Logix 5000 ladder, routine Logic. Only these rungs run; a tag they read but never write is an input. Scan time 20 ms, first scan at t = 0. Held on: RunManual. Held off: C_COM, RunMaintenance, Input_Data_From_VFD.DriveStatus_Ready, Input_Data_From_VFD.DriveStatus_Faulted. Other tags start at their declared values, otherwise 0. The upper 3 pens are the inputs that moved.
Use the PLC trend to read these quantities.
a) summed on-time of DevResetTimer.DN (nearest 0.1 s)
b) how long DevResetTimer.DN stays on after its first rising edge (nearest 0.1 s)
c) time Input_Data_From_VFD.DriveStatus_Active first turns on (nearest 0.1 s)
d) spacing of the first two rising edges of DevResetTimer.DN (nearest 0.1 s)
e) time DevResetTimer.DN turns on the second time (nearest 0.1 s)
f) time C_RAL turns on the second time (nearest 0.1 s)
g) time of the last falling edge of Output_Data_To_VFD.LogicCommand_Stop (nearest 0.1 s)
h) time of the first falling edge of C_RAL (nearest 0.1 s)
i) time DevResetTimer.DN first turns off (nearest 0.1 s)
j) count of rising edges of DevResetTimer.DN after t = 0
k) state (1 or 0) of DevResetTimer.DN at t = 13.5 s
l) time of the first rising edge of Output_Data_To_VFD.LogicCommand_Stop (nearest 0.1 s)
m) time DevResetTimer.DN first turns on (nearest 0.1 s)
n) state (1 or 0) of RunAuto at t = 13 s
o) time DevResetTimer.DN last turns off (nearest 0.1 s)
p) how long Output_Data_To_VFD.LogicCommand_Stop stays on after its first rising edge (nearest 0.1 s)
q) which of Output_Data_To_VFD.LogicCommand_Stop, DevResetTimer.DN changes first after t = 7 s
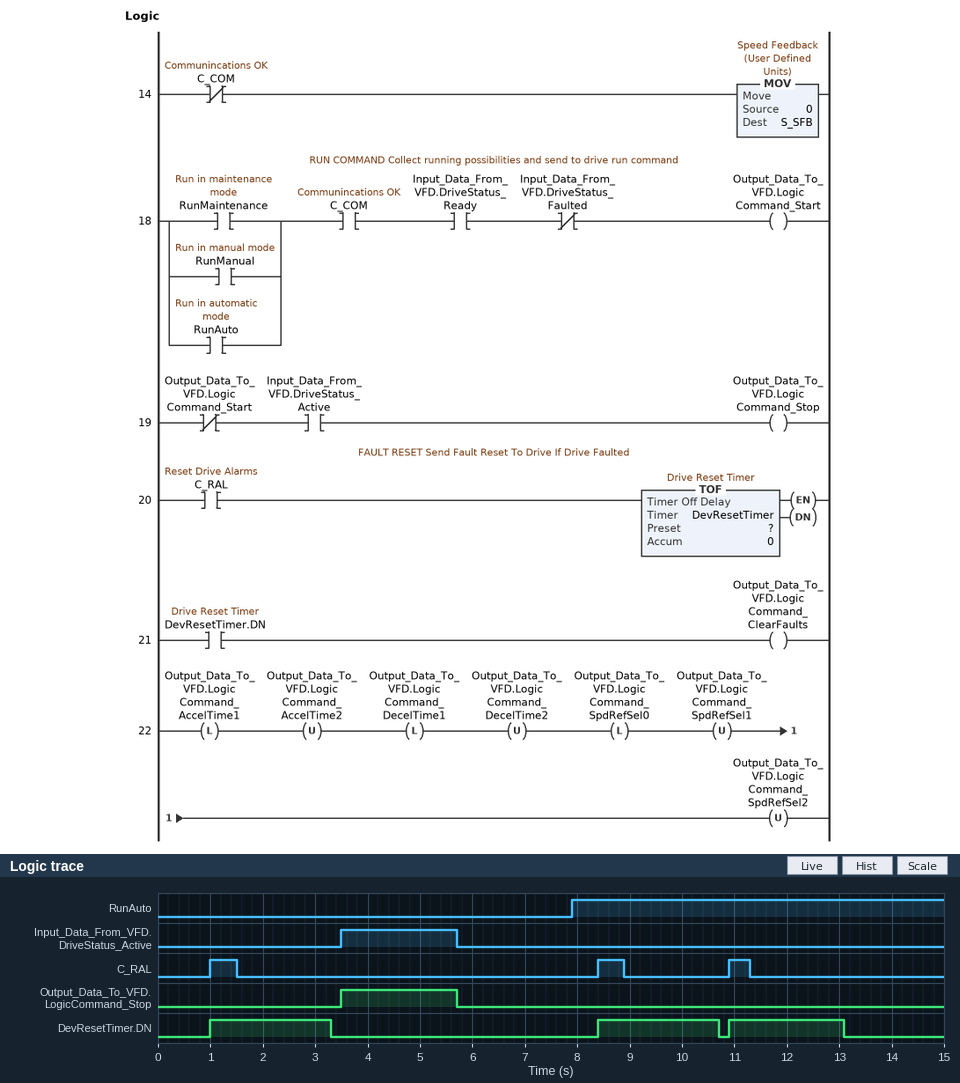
6.8 s
2.3 s
3.5 s
7.4 s
8.4 s
8.4 s
5.7 s
1.5 s
3.3 s
3
0
3.5 s
1.0 s
1
13.1 s
2.2 s
DevResetTimer.DN
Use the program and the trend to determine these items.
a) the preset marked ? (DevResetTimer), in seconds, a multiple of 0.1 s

1.8 s
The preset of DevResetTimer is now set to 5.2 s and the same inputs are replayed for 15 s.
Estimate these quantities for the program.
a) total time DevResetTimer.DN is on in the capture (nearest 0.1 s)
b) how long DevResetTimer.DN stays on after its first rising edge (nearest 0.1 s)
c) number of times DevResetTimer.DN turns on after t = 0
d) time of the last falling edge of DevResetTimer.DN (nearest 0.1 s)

12.3 s
5.7 s
2
6.7 s
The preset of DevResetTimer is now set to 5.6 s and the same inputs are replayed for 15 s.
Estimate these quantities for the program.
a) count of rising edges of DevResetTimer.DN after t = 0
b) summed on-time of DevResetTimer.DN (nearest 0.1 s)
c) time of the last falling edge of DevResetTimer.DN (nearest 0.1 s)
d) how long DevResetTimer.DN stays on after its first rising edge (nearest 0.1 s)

2
12.7 s
7.1 s
6.1 s
